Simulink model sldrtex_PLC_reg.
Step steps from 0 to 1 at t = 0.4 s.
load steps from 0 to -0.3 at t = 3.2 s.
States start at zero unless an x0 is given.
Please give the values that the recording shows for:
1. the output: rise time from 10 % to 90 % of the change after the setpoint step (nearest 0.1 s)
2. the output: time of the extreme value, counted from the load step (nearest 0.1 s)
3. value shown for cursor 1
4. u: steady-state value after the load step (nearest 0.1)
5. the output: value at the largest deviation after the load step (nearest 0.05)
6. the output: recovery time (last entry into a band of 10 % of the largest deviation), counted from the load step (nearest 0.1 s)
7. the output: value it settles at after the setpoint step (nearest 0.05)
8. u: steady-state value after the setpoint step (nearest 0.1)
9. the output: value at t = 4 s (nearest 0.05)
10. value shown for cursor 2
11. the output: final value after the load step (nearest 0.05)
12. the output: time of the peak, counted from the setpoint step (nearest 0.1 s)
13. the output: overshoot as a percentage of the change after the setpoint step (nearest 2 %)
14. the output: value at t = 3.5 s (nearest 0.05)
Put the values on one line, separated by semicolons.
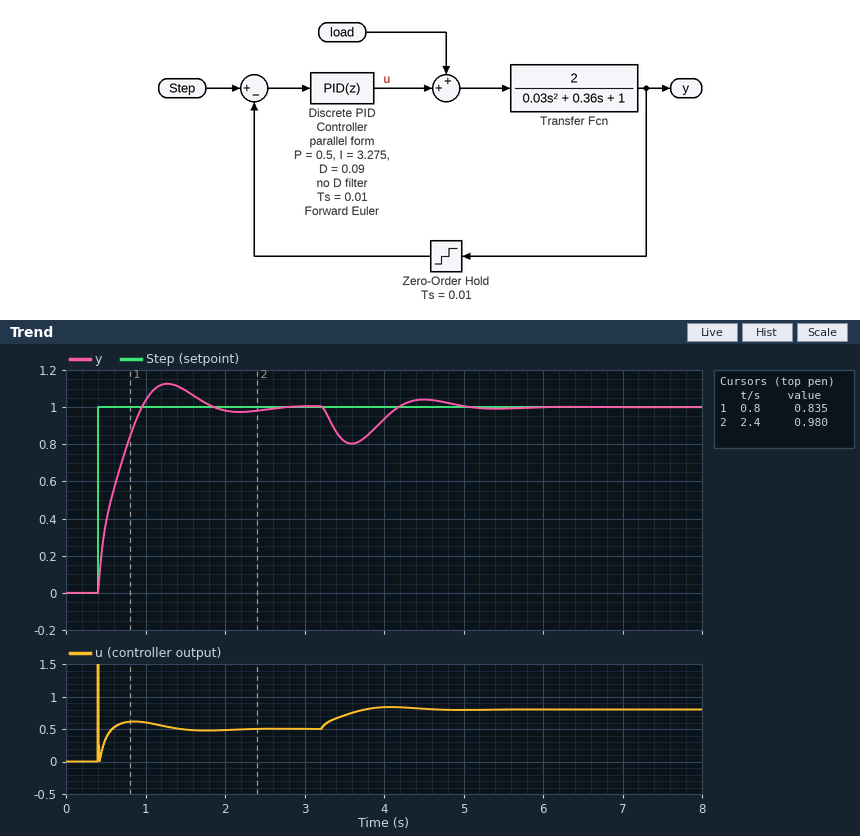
0.4 s; 0.4 s; 0.835; 0.8; 0.80; 1.6 s; 1.00; 0.5; 0.95; 0.980; 1.00; 0.9 s; 12 %; 0.80
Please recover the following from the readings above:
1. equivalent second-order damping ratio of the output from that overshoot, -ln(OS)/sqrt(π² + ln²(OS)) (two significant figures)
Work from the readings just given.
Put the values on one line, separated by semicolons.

0.56
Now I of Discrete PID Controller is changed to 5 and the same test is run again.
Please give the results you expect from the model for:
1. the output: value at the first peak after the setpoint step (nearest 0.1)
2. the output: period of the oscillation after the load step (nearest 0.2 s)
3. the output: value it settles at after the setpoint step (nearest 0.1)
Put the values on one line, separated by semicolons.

1.2; 1.4 s; 1.0
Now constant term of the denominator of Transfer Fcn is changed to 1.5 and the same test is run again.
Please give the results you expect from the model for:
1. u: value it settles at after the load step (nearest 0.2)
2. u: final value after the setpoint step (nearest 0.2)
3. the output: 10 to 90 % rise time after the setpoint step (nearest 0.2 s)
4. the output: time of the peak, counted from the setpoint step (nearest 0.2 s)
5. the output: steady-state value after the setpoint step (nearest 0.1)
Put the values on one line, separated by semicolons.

1.0; 0.8; 0.6 s; 1.0 s; 1.0
